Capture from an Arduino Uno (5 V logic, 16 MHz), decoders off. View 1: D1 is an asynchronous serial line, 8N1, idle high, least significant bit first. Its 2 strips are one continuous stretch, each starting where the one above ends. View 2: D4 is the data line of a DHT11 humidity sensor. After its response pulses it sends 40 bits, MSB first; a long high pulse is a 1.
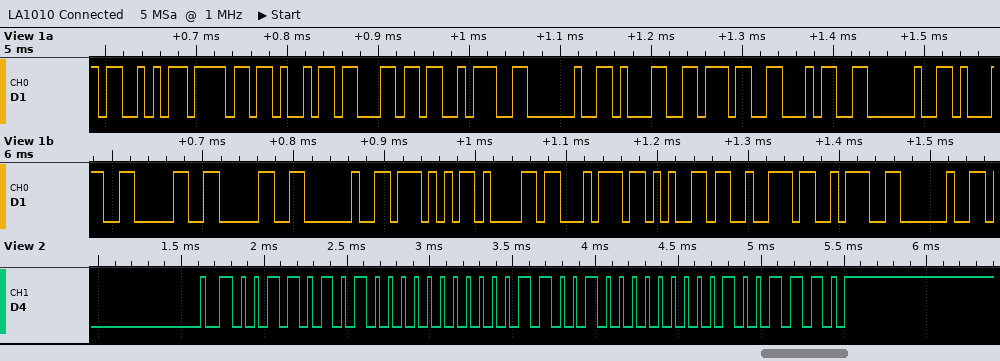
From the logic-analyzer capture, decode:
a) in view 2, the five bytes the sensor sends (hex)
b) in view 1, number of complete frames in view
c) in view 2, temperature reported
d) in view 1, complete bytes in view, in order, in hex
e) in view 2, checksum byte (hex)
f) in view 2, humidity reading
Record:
35 00 19 00 4E
21
25.0 °C
53 6F 69 6C 3A 20 31 37 34 20 31 30 30 20 57 61 74 65 72 3A 20
0x4E
53 %
